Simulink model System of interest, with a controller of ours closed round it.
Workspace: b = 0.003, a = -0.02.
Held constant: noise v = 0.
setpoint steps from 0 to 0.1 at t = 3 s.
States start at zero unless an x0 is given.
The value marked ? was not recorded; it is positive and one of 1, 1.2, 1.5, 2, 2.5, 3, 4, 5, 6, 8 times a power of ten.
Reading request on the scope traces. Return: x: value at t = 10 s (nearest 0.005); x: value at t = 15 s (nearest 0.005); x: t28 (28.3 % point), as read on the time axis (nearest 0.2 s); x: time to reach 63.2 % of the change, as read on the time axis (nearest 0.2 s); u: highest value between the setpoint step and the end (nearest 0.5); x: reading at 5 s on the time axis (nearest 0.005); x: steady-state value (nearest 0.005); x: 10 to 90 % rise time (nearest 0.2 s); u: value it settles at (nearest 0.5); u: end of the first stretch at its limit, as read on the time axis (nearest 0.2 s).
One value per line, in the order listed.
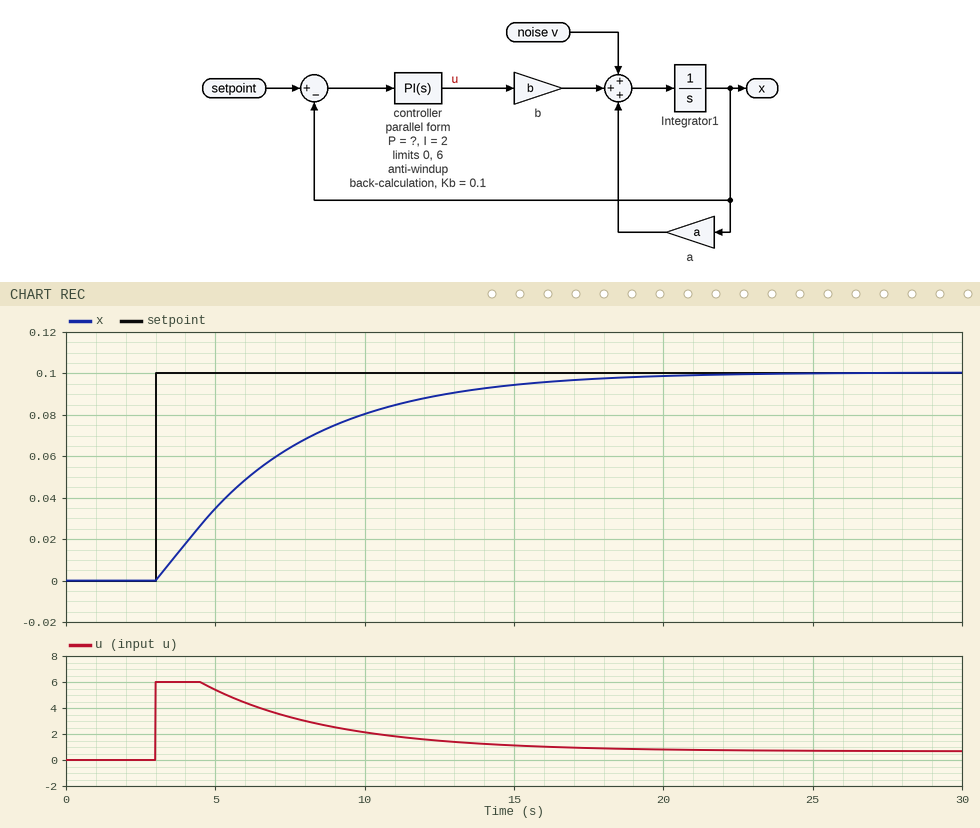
0.080
0.095
4.6 s
7.4 s
6.0
0.035
0.100
9.2 s
0.5
4.6 s
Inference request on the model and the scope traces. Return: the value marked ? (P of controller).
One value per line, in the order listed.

80
